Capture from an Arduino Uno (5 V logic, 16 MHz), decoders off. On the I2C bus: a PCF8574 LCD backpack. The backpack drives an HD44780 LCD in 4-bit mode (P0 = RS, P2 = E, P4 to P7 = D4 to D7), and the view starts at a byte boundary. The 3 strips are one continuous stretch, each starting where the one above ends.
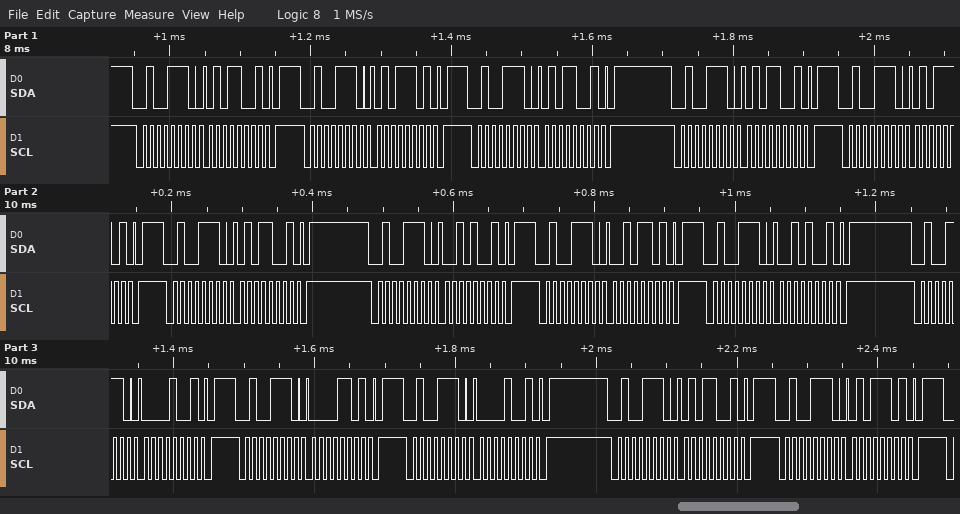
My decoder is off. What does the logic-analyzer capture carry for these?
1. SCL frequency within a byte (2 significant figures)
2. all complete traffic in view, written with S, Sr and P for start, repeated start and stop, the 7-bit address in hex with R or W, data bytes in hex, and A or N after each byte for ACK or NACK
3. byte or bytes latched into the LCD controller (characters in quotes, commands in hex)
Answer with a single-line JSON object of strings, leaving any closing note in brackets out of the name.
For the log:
{"SCL frequency within a byte": "100 kHz", "all complete traffic in view, written with S, Sr and P for start, repeated start and stop, the 7-bit address in hex with R or W, data bytes in hex, and A or N after each byte for ACK or NACK": "S 27W A 59 A P S 27W A 5D A P S 27W A 59 A P S 27W A 59 A P S 27W A 5D A P S 27W A 59 A P S 27W A 29 A P S 27W A 2D A P S 27W A 29 A P S 27W A 09 A P S 27W A 0D A P S 27W A 09 A P S 27W A 59 A P S 27W A 5D A P", "byte or bytes latched into the LCD controller": "'U' ' '"}
